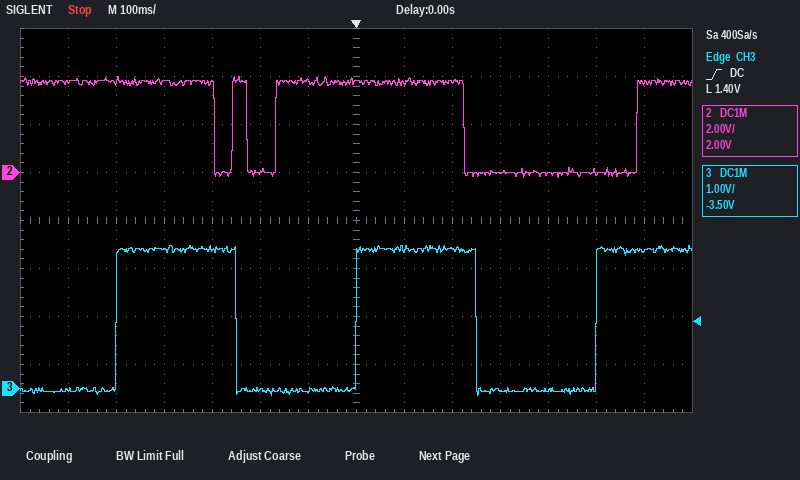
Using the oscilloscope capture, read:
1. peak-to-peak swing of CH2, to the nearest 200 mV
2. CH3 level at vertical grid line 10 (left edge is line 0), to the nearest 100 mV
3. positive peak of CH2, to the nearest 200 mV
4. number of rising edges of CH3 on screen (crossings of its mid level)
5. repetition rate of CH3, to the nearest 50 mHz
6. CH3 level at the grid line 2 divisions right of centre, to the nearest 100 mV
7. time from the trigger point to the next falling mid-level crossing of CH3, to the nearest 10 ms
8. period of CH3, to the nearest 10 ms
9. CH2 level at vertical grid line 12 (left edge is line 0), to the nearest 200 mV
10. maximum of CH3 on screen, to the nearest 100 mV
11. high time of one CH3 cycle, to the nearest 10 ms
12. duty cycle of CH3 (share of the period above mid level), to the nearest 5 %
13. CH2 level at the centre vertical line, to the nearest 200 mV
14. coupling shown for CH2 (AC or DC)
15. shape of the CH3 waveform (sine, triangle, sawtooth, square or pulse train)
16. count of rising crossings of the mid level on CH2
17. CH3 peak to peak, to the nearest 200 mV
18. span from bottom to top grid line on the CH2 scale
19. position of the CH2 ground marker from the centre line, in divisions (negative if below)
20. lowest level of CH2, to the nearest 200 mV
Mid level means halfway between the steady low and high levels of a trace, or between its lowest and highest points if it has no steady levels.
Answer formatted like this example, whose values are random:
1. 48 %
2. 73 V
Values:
1. 4.2 V
2. 0.0 V
3. 4.0 V
4. 3
5. 2.00 Hz
6. 2.9 V
7. 250 ms
8. 500 ms
9. 0.0 V
10. 3.0 V
11. 250 ms
12. 50 %
13. 3.8 V
14. DC
15. square
16. 3
17. 3.2 V
18. 16 V
19. +1.0 div
20. -200 mV
